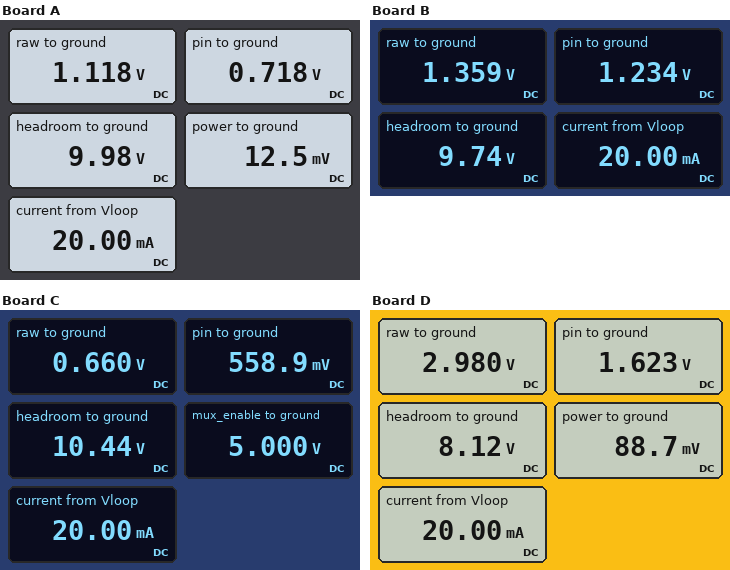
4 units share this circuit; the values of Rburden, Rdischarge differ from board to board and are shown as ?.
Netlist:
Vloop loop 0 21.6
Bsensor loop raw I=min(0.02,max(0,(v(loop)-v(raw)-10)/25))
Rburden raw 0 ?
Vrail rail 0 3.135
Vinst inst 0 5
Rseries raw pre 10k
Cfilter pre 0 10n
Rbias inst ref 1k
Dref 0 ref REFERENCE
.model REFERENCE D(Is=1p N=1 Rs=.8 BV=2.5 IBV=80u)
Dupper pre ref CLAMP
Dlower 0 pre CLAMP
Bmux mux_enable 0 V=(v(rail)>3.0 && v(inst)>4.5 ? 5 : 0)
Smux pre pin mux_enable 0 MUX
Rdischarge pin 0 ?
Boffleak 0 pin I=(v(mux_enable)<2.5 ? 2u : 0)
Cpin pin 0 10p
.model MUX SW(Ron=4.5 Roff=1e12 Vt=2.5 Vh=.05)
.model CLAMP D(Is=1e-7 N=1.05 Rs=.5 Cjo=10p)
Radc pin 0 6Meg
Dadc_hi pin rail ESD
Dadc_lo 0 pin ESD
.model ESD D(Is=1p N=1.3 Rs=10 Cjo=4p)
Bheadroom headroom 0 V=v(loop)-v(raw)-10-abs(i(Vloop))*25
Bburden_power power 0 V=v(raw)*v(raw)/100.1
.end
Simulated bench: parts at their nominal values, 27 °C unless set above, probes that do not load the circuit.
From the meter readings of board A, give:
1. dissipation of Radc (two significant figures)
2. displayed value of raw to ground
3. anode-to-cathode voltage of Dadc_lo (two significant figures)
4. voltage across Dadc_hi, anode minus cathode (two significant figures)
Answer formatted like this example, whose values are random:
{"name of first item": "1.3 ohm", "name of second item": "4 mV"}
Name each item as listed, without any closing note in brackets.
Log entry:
{"dissipation of Radc": "86 nW", "displayed value of raw to ground": "1.118 V", "anode-to-cathode voltage of Dadc_lo": "-720 mV", "voltage across Dadc_hi, anode minus cathode": "-2.4 V"}
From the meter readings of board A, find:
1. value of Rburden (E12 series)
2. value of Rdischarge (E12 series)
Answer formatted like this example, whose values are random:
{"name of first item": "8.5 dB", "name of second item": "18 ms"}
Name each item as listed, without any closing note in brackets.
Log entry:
{"value of Rburden": "56 Ω", "value of Rdischarge": "18 kΩ"}
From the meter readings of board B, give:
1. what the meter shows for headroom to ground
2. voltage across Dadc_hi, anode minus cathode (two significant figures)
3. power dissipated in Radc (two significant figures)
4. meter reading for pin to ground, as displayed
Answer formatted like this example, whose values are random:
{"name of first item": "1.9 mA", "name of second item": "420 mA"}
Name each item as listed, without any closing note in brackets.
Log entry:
{"what the meter shows for headroom to ground": "9.74 V", "voltage across Dadc_hi, anode minus cathode": "-1.9 V", "power dissipated in Radc": "250 nW", "meter reading for pin to ground, as displayed": "1.234 V"}
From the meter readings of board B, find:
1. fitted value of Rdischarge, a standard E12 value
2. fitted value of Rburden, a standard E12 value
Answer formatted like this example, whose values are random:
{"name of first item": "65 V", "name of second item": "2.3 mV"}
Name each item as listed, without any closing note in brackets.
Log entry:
{"fitted value of Rdischarge, a standard E12 value": "100 kΩ", "fitted value of Rburden, a standard E12 value": "68 Ω"}
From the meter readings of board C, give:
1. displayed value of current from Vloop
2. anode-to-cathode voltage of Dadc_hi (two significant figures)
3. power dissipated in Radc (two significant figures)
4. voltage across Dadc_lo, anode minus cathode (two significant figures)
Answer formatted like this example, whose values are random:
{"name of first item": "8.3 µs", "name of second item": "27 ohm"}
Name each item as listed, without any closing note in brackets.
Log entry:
{"displayed value of current from Vloop": "20.00 mA", "anode-to-cathode voltage of Dadc_hi": "-2.6 V", "power dissipated in Radc": "52 nW", "voltage across Dadc_lo, anode minus cathode": "-560 mV"}
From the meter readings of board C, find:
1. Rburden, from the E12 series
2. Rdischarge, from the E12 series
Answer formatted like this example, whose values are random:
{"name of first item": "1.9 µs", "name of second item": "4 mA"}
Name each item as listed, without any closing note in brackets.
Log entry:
{"Rburden, from the E12 series": "33 Ω", "Rdischarge, from the E12 series": "56 kΩ"}
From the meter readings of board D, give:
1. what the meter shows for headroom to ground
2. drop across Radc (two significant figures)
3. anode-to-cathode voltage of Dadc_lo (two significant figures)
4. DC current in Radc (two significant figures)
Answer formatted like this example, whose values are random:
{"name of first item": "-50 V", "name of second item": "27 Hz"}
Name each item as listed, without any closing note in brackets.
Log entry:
{"what the meter shows for headroom to ground": "8.12 V", "drop across Radc": "1.6 V", "anode-to-cathode voltage of Dadc_lo": "-1.6 V", "DC current in Radc": "270 nA"}
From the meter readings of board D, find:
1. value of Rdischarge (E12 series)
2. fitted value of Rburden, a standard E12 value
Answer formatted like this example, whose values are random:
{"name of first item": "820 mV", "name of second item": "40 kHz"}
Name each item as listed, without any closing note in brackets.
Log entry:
{"value of Rdischarge": "12 kΩ", "fitted value of Rburden, a standard E12 value": "150 Ω"}
